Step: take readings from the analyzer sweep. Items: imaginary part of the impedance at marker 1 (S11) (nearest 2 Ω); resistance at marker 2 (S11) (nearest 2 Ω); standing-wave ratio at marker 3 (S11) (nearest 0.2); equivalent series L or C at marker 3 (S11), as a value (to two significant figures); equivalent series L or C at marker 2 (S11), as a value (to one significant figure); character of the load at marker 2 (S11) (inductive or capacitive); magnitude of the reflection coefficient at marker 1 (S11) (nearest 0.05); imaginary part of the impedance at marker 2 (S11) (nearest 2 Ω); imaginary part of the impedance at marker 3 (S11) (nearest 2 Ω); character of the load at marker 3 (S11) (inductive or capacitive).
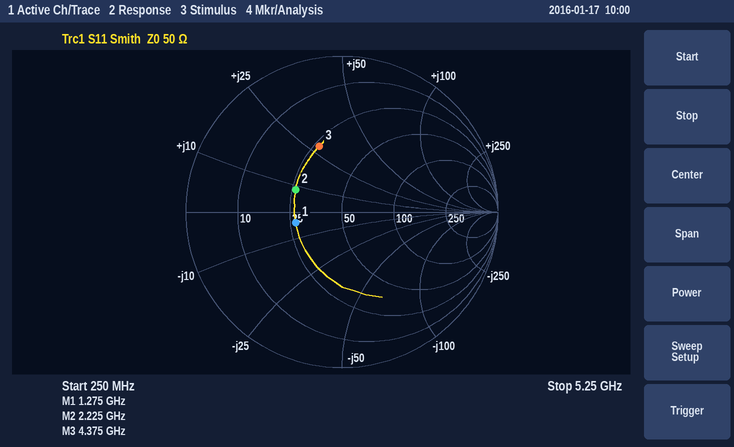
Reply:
-4 Ω
26 Ω
2.6
1.0 nH
600 pH
inductive
0.30
+8 Ω
+28 Ω
inductive
